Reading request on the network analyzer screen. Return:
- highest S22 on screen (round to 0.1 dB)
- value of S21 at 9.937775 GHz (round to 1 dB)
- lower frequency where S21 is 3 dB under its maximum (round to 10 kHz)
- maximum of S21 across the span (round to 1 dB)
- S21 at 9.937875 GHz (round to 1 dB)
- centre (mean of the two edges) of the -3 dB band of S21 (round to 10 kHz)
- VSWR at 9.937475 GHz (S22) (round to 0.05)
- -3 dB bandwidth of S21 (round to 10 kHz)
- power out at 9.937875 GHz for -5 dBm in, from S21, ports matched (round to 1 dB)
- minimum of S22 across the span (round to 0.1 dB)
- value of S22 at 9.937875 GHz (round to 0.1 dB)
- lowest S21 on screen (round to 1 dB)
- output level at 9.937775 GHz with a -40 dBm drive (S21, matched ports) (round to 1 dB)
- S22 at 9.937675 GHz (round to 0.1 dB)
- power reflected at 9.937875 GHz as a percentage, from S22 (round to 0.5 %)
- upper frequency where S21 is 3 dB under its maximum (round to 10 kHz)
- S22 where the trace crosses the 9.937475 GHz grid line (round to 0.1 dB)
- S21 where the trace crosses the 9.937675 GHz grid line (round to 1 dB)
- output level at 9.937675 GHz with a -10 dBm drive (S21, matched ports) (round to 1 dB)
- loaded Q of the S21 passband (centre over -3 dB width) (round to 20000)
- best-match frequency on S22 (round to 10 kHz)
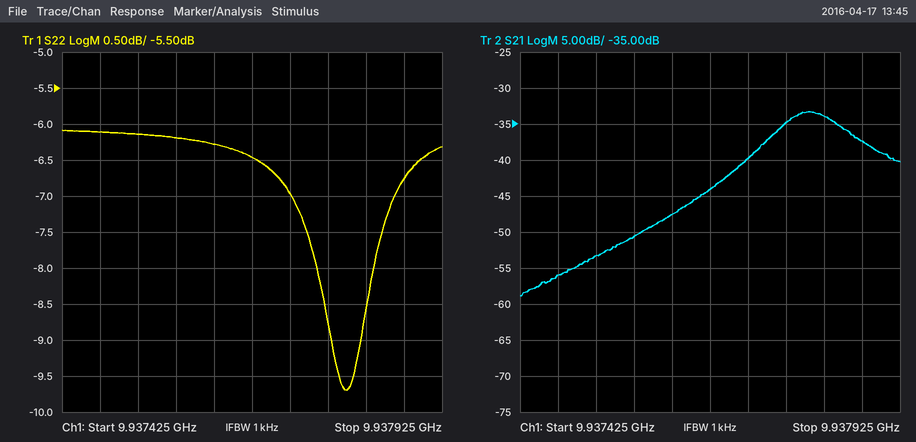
-6.1 dB
-35 dB
9.93776 GHz
-33 dB
-37 dB
9.93781 GHz
2.95
100 kHz
-42 dBm
-9.7 dB
-6.8 dB
-59 dB
-75 dBm
-6.5 dB
21.0 %
9.93786 GHz
-6.1 dB
-44 dB
-54 dBm
100000
9.93780 GHz
